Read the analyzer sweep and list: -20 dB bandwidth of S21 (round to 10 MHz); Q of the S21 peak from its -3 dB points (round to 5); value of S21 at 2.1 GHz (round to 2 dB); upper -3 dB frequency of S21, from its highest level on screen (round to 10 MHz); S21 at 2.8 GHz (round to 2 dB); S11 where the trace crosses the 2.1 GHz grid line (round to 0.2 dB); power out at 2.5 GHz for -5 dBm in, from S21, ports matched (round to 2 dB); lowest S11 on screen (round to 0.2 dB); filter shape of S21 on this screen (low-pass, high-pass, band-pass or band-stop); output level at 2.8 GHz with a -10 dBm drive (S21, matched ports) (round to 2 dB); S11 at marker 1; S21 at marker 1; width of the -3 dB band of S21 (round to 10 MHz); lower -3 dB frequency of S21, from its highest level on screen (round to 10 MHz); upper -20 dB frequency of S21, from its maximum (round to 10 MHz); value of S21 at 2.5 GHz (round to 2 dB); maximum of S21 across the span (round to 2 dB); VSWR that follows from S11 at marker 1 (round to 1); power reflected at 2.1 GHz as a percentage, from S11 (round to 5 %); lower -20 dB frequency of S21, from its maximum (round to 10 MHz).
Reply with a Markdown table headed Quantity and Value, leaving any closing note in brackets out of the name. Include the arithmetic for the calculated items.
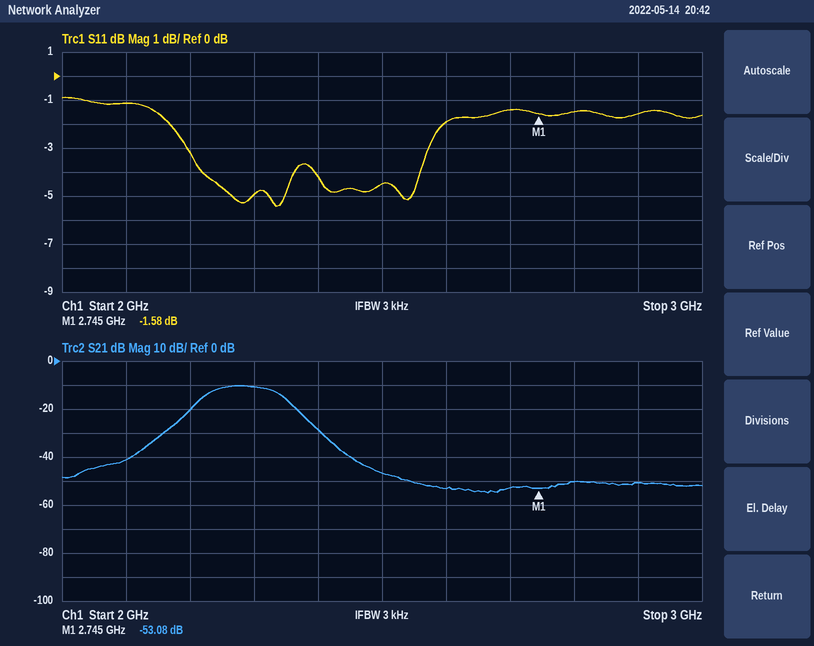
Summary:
| Quantity | Value |
|---|---|
| -20 dB bandwidth of S21 | 2.41 GHz − 2.16 GHz = 250 MHz |
| Q of the S21 peak from its -3 dB points | 2.285 GHz / 110 MHz ≈ 20.8, so 20 to the nearest 5 |
| value of S21 at 2.1 GHz | -42 dB |
| upper -3 dB frequency of S21, from its highest level on screen | 2.34 GHz |
| S21 at 2.8 GHz | -50 dB |
| S11 where the trace crosses the 2.1 GHz grid line | -1.2 dB |
| power out at 2.5 GHz for -5 dBm in, from S21, ports matched | -5 dBm + (-46 dB) = -52 dBm |
| lowest S11 on screen | -5.4 dB |
| filter shape of S21 on this screen | band-pass |
| output level at 2.8 GHz with a -10 dBm drive (S21, matched ports) | -10 dBm + (-50 dB) = -60 dBm |
| S11 at marker 1 | -1.58 dB |
| S21 at marker 1 | -53.08 dB |
| width of the -3 dB band of S21 | 2.34 GHz − 2.23 GHz = 110 MHz |
| lower -3 dB frequency of S21, from its highest level on screen | 2.23 GHz |
| upper -20 dB frequency of S21, from its maximum | 2.41 GHz |
| value of S21 at 2.5 GHz | -46 dB |
| maximum of S21 across the span | -10 dB |
| VSWR that follows from S11 at marker 1 | (1 + 0.8337)/(1 − 0.8337) ≈ 11 |
| power reflected at 2.1 GHz as a percentage, from S11 | 10^(-1.2/10) ≈ 75.9 %, so 75 % to the nearest 5 % |
| lower -20 dB frequency of S21, from its maximum | 2.16 GHz |
